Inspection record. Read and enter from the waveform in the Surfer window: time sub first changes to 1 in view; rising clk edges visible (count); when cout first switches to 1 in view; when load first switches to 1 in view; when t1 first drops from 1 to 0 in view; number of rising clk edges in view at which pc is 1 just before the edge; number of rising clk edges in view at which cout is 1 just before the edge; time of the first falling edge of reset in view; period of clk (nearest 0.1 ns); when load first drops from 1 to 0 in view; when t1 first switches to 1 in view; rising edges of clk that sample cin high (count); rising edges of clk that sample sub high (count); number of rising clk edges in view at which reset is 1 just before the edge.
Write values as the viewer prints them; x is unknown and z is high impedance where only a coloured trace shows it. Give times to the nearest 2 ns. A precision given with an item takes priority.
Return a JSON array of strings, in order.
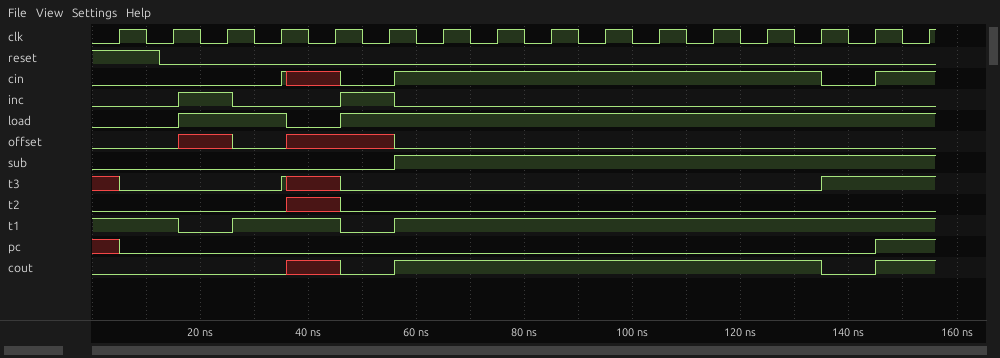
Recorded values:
["56 ns", "16", "56 ns", "16 ns", "16 ns", "1", "9", "12 ns", "10 ns", "36 ns", "26 ns", "9", "10", "1"]
